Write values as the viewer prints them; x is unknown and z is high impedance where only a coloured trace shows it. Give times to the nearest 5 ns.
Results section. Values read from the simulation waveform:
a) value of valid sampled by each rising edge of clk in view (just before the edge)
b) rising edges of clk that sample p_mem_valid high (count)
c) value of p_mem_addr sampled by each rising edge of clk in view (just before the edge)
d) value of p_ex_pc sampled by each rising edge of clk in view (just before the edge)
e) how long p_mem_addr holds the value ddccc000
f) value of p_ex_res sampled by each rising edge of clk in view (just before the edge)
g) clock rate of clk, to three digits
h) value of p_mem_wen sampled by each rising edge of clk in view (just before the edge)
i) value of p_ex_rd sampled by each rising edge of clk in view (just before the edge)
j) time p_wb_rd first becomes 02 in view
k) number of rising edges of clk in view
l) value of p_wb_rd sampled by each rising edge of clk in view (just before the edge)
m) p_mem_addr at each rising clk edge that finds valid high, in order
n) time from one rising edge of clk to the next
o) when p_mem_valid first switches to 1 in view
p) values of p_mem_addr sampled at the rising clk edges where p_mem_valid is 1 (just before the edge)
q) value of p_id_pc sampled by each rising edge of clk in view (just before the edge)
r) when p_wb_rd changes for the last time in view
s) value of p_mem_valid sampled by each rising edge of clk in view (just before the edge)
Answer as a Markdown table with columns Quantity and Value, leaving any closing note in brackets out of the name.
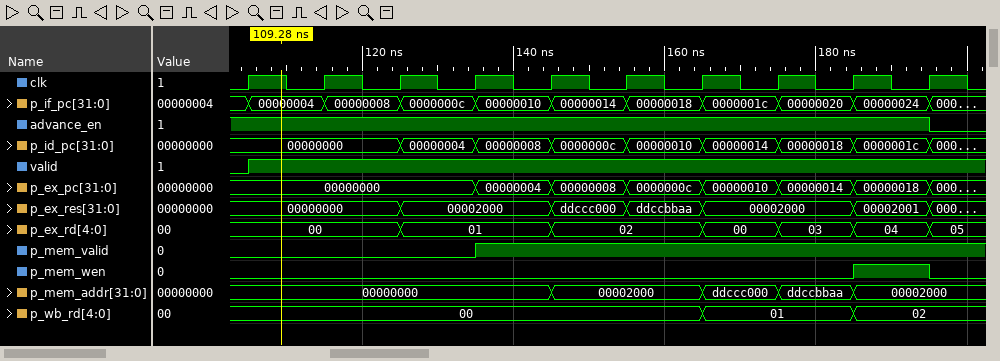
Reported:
| Quantity | Value |
|---|---|
| value of valid sampled by each rising edge of clk in view | 0 1 1 1 1 1 1 1 1 1 |
| rising edges of clk that sample p_mem_valid high | 6 |
| value of p_mem_addr sampled by each rising edge of clk in view | 00000000, 00000000, 00000000, 00000000, 00000000, 00002000, 00002000, ddccc000, ddccbbaa, 00002000 |
| value of p_ex_pc sampled by each rising edge of clk in view | 00000000, 00000000, 00000000, 00000000, 00000004, 00000008, 0000000c, 00000010, 00000014, 00000018 |
| how long p_mem_addr holds the value ddccc000 | 10 ns |
| value of p_ex_res sampled by each rising edge of clk in view | 00000000, 00000000, 00000000, 00002000, 00002000, ddccc000, ddccbbaa, 00002000, 00002000, 00002001 |
| clock rate of clk, to three digits | 100 MHz |
| value of p_mem_wen sampled by each rising edge of clk in view | 0 0 0 0 0 0 0 0 0 1 |
| value of p_ex_rd sampled by each rising edge of clk in view | 00, 00, 00, 01, 01, 02, 02, 00, 03, 04 |
| time p_wb_rd first becomes 02 in view | 185 ns |
| number of rising edges of clk in view | 10 |
| value of p_wb_rd sampled by each rising edge of clk in view | 00, 00, 00, 00, 00, 00, 00, 01, 01, 02 |
| p_mem_addr at each rising clk edge that finds valid high, in order | 00000000, 00000000, 00000000, 00000000, 00002000, 00002000, ddccc000, ddccbbaa, 00002000 |
| time from one rising edge of clk to the next | 10 ns |
| when p_mem_valid first switches to 1 in view | 135 ns |
| values of p_mem_addr sampled at the rising clk edges where p_mem_valid is 1 | 00000000, 00002000, 00002000, ddccc000, ddccbbaa, 00002000 |
| value of p_id_pc sampled by each rising edge of clk in view | 00000000, 00000000, 00000000, 00000004, 00000008, 0000000c, 00000010, 00000014, 00000018, 0000001c |
| when p_wb_rd changes for the last time in view | 185 ns |
| value of p_mem_valid sampled by each rising edge of clk in view | 0 0 0 0 1 1 1 1 1 1 |
